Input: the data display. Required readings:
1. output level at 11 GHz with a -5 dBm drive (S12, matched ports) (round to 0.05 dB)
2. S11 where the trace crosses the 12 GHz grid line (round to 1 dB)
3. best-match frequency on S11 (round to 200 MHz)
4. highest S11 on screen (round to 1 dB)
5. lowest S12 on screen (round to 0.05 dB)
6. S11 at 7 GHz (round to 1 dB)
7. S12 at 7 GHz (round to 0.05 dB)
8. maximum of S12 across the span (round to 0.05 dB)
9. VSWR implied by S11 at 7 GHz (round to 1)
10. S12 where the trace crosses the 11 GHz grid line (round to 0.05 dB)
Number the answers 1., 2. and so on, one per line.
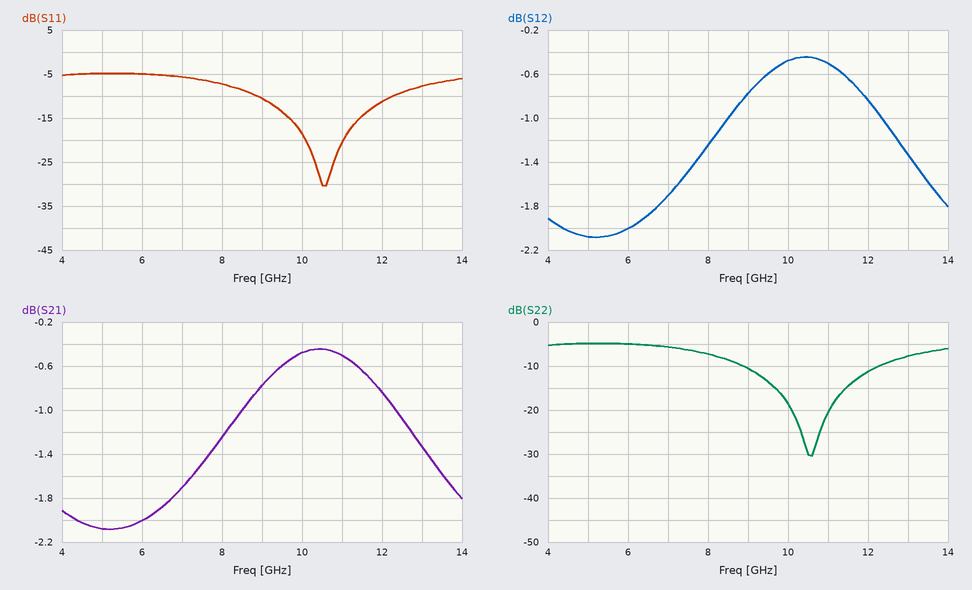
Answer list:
1. -5.50 dBm
2. -11 dB
3. 10.6 GHz
4. -5 dB
5. -2.10 dB
6. -6 dB
7. -1.70 dB
8. -0.45 dB
9. 3
10. -0.50 dB
